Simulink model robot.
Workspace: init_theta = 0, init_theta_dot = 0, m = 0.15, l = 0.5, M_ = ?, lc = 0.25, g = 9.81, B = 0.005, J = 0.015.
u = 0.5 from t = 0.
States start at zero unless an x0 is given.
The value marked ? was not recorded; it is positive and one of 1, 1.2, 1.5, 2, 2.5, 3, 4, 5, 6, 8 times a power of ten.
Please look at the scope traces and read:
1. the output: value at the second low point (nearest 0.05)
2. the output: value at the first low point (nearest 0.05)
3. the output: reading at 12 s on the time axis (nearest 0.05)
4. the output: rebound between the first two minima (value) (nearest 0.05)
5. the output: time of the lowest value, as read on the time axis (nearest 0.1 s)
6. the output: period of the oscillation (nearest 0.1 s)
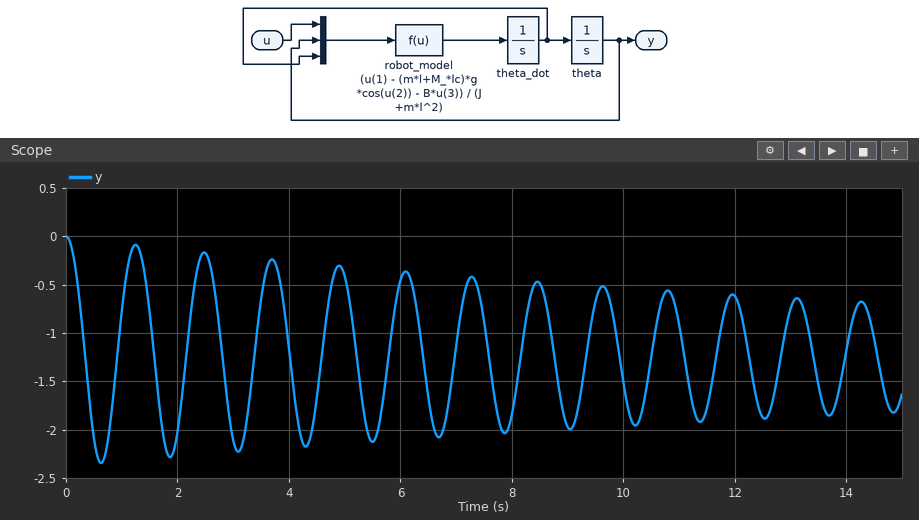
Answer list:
-2.30
-2.35
-0.60
-0.10
0.6 s
1.2 s
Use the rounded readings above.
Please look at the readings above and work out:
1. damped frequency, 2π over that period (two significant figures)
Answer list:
5.2 rad/s
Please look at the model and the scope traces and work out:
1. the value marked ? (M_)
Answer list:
0.4
